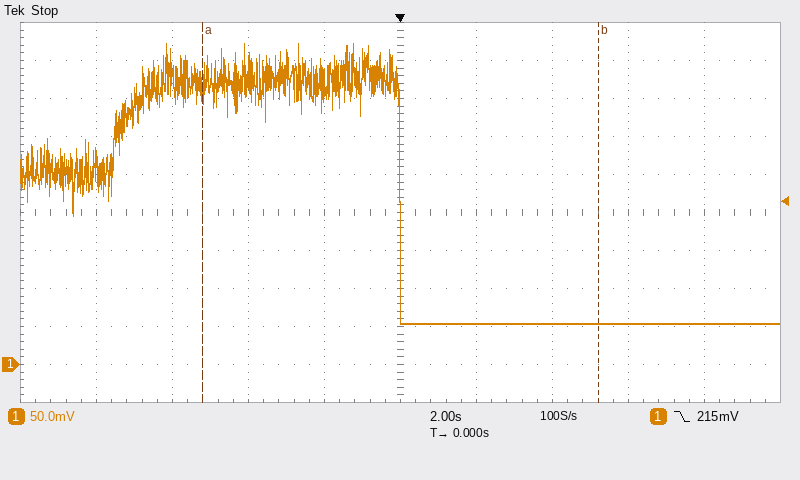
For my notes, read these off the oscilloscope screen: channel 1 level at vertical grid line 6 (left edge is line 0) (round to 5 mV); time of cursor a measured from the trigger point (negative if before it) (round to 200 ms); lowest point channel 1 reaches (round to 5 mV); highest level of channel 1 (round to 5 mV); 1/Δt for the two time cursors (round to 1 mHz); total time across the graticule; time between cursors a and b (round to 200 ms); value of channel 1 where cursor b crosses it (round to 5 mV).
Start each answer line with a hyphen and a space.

- 55 mV
- -5.2 s
- 55 mV
- 420 mV
- 96 mHz
- 20 s
- 10.4 s
- 55 mV
